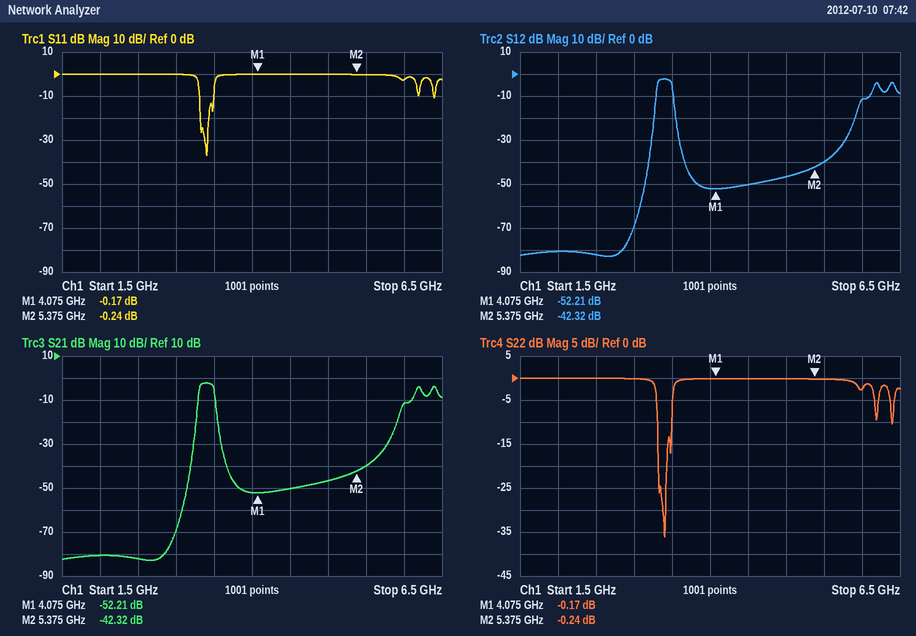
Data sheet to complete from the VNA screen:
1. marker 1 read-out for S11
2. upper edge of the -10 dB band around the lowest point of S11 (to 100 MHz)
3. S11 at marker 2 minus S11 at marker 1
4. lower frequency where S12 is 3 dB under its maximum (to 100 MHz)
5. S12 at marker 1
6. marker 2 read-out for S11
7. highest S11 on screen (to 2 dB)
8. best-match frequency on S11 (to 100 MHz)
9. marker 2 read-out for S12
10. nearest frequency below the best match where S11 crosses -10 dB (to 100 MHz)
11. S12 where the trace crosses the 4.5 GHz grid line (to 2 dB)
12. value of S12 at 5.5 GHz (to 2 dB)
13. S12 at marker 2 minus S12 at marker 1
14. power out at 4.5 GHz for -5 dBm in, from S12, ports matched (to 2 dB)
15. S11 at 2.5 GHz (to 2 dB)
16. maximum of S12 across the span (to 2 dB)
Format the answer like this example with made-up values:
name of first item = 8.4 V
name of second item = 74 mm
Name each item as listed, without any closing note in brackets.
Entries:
marker 1 read-out for S11 = -0.17 dB
upper edge of the -10 dB band around the lowest point of S11 = 3.5 GHz
S11 at marker 2 minus S11 at marker 1 = -0.07 dB
lower frequency where S12 is 3 dB under its maximum = 3.3 GHz
S12 at marker 1 = -52.21 dB
marker 2 read-out for S11 = -0.24 dB
highest S11 on screen = 0 dB
best-match frequency on S11 = 3.4 GHz
marker 2 read-out for S12 = -42.32 dB
nearest frequency below the best match where S11 crosses -10 dB = 3.3 GHz
S12 where the trace crosses the 4.5 GHz grid line = -50 dB
value of S12 at 5.5 GHz = -40 dB
S12 at marker 2 minus S12 at marker 1 = 9.89 dB
power out at 4.5 GHz for -5 dBm in, from S12, ports matched = -56 dBm
S11 at 2.5 GHz = 0 dB
maximum of S12 across the span = -2 dB
